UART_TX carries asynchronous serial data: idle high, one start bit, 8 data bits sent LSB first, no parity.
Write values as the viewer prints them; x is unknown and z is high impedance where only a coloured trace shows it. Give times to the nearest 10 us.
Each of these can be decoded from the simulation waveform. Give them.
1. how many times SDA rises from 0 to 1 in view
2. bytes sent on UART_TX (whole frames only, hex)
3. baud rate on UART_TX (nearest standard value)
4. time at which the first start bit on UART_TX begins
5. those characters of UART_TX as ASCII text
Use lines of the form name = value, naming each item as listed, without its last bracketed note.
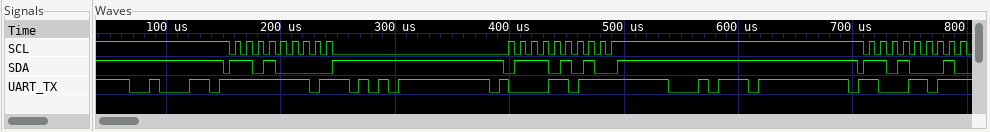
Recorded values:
how many times SDA rises from 0 to 1 in view = 10
bytes sent on UART_TX = 62, 57, 61, 74, 63
baud rate on UART_TX = 115200 baud
time at which the first start bit on UART_TX begins = 70 us
those characters of UART_TX as ASCII text = "bWatc"
